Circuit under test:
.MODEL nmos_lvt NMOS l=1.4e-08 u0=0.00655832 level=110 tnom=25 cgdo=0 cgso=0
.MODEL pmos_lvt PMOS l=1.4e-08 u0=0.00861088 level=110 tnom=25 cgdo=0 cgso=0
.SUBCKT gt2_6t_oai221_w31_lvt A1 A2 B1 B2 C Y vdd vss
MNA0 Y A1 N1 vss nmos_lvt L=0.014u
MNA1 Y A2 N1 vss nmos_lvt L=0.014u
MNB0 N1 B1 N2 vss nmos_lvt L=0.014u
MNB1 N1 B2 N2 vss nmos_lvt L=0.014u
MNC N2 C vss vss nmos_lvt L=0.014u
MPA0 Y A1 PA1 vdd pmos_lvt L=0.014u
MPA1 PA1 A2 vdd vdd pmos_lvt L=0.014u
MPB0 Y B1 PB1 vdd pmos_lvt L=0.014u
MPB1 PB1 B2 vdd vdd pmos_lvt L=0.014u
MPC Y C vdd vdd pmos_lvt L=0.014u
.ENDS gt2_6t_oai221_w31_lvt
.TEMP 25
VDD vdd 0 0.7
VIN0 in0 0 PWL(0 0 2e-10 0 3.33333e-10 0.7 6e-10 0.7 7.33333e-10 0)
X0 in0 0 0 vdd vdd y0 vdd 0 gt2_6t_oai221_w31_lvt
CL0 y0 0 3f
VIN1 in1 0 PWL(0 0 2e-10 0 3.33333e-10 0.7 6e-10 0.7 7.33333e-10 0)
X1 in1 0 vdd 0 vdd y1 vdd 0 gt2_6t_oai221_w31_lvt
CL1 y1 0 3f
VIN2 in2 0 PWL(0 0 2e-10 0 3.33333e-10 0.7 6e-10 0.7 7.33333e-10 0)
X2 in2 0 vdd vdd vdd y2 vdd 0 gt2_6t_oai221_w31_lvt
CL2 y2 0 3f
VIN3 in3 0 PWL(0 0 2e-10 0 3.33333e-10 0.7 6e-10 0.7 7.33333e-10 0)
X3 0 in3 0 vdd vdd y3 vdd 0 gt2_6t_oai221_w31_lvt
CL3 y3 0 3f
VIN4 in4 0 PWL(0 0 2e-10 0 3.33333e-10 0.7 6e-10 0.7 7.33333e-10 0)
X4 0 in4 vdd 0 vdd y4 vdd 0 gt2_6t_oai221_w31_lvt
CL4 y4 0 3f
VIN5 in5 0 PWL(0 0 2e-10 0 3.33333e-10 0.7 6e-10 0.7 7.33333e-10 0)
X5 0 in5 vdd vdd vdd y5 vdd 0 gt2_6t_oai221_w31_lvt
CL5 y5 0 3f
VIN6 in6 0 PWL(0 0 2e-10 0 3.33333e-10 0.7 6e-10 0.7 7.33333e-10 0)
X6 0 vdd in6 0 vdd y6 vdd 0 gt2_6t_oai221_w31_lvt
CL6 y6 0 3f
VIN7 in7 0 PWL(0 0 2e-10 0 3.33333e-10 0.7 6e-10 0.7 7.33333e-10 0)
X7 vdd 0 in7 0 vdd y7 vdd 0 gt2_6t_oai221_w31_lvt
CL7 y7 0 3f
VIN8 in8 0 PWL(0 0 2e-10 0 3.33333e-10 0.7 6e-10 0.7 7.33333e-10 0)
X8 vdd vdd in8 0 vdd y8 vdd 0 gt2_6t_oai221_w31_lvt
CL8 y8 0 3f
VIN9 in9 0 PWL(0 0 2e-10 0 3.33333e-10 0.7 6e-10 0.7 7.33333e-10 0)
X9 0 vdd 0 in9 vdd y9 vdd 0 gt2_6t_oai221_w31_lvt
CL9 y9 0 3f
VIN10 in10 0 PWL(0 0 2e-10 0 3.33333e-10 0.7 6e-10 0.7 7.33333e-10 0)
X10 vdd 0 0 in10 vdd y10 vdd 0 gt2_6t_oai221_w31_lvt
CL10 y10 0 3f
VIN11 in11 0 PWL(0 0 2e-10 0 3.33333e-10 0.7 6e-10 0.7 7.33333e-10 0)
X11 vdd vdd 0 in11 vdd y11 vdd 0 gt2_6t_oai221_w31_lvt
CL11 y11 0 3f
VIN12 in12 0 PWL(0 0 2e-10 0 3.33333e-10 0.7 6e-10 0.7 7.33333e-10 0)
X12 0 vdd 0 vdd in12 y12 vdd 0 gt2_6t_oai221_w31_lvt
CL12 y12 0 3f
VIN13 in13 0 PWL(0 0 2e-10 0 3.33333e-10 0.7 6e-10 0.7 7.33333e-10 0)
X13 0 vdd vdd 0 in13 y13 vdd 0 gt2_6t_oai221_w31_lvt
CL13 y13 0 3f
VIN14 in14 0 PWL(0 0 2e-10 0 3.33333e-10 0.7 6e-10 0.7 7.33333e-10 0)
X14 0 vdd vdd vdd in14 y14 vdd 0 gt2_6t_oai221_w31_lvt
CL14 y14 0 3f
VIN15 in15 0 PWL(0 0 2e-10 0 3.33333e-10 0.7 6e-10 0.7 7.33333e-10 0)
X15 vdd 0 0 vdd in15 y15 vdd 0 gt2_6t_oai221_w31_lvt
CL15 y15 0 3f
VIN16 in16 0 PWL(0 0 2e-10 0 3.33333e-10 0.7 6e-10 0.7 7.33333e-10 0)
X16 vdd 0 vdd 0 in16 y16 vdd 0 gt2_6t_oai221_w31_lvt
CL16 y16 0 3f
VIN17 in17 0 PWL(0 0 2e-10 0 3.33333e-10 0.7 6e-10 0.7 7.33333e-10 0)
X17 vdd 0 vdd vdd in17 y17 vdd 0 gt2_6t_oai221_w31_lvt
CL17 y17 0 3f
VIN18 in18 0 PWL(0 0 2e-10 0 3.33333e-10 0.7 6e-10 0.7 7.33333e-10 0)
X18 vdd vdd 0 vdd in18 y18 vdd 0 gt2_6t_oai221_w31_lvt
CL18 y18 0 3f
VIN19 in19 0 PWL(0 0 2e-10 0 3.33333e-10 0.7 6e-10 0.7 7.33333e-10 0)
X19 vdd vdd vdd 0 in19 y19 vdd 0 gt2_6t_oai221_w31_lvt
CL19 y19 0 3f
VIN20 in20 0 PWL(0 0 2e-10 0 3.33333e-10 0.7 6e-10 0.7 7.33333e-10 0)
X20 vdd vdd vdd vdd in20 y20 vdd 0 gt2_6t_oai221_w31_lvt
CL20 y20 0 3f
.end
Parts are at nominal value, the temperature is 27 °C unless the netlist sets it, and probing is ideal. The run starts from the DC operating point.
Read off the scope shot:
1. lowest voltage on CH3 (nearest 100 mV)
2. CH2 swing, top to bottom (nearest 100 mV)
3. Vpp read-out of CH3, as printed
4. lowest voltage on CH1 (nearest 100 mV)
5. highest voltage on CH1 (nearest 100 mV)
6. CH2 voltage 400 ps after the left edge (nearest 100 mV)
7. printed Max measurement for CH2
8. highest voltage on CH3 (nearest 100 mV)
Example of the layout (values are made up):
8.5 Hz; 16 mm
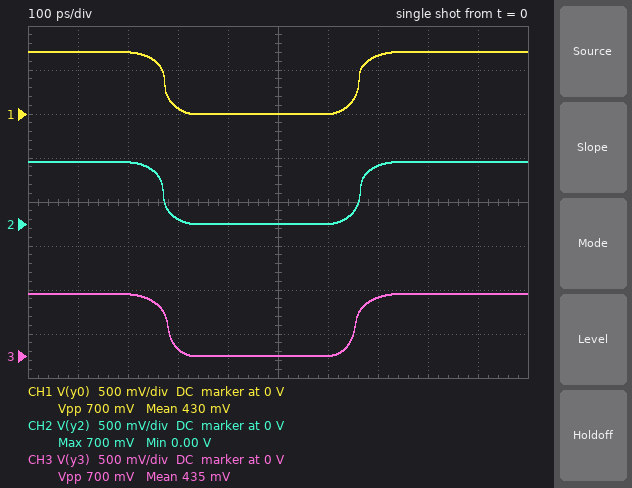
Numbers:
0 V; 700 mV; 700 mV; 0 V; 700 mV; 0 V; 700 mV; 700 mV
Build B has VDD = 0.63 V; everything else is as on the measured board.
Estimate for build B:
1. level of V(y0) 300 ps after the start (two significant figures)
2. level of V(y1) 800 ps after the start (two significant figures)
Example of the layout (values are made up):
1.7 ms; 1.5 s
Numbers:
25 mV; 630 mV
